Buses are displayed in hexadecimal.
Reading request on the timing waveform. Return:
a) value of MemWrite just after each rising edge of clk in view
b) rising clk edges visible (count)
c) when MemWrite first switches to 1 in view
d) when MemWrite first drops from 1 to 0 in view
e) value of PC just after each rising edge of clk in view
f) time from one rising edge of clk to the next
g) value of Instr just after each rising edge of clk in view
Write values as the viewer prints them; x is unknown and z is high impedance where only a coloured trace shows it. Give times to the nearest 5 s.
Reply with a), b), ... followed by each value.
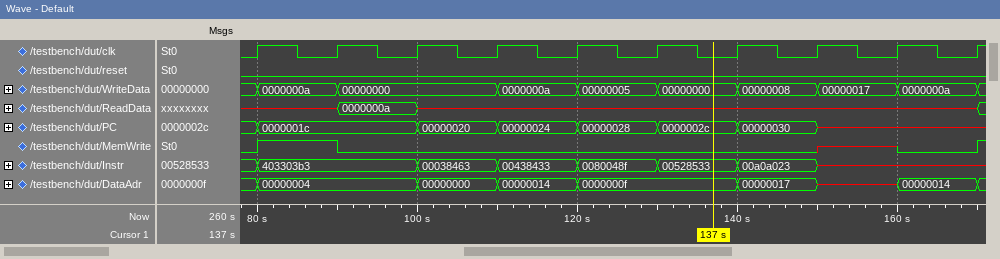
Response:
a) 1 0 0 0 0 0 0 x 0 1
b) 10
c) 80 s
d) 90 s
e) 0000001c, 0000001c, 00000020, 00000024, 00000028, 0000002c, 00000030, x, x, x
f) 10 s
g) 403303b3, 403303b3, 00038463, 00438433, 0080048f, 00528533, 00a0a023, x, x, x
